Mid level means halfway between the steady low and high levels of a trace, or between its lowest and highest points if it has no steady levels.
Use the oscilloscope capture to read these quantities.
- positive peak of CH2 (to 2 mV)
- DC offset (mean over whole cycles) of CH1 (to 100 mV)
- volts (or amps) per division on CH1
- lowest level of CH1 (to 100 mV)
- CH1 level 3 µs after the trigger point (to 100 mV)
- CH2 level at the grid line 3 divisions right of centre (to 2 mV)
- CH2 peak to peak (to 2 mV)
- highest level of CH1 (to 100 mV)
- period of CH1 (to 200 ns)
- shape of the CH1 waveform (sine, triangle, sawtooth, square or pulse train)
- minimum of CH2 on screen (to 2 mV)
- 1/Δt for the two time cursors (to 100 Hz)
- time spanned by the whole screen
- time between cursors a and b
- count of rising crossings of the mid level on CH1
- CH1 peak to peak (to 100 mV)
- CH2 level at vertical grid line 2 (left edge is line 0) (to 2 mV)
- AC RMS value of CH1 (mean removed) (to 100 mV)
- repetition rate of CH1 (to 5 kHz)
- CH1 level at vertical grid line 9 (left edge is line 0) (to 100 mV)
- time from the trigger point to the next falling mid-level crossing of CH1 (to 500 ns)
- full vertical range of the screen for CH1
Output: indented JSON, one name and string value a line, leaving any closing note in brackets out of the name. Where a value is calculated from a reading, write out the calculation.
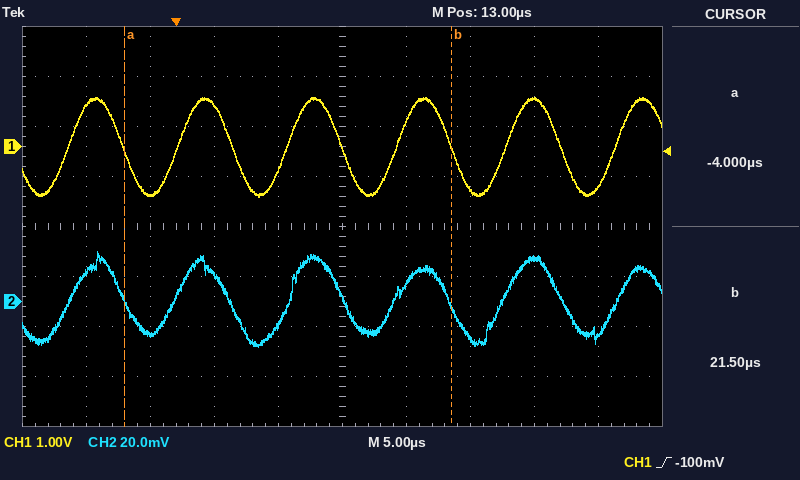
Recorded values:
{
  "positive peak of CH2": "20 mV",
  "DC offset (mean over whole cycles) of CH1": "(1.0 V + (-1.0 V)) / 2 ≈ 0.0 V",
  "volts (or amps) per division on CH1": "1 V",
  "lowest level of CH1": "-1.0 V",
  "CH1 level 3 µs after the trigger point": "800 mV",
  "CH2 level at the grid line 3 divisions right of centre": "18 mV",
  "CH2 peak to peak": "20 mV − (-18 mV) = 38 mV",
  "highest level of CH1": "1.0 V",
  "period of CH1": "8.6 µs",
  "shape of the CH1 waveform": "sine",
  "minimum of CH2 on screen": "-18 mV",
  "1/Δt for the two time cursors": "1 / 25.5 µs ≈ 39.2 kHz",
  "time spanned by the whole screen": "50 µs",
  "time between cursors a and b": "21.5 µs − (-4 µs) = 25.5 µs",
  "count of rising crossings of the mid level on CH1": "6",
  "CH1 peak to peak": "1.0 V − (-1.0 V) = 2.0 V",
  "CH2 level at vertical grid line 2 (left edge is line 0)": "-12 mV",
  "AC RMS value of CH1 (mean removed)": "2.0 V / (2√2) ≈ 707 mV, so 700 mV to the nearest 100 mV",
  "repetition rate of CH1": "1 / 8.6 µs ≈ 116 kHz, so 115 kHz to the nearest 5 kHz",
  "CH1 level at vertical grid line 9 (left edge is line 0)": "-800 mV",
  "time from the trigger point to the next falling mid-level crossing of CH1": "4.5 µs",
  "full vertical range of the screen for CH1": "8 V"
}
